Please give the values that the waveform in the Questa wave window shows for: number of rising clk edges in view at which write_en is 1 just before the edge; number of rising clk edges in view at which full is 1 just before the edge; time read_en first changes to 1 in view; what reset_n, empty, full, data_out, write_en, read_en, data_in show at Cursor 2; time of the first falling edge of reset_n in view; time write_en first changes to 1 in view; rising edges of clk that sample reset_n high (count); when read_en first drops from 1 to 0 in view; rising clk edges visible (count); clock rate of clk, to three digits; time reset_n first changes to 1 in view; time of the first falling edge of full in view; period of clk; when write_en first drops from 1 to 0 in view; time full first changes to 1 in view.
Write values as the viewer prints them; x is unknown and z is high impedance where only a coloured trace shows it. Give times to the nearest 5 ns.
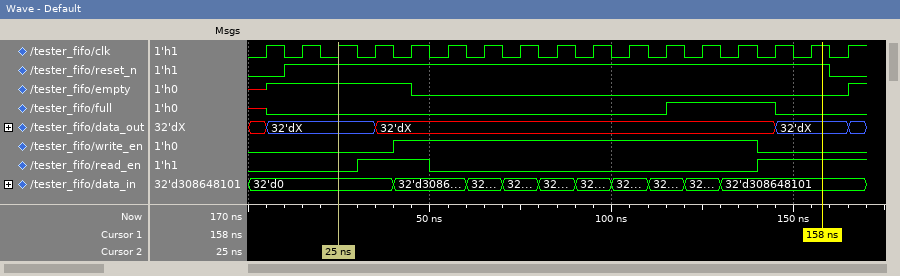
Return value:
10
3
30 ns
reset_n=1, empty=1, full=0, data_out=32'dX, write_en=0, read_en=0, data_in=32'd0
160 ns
40 ns
15
50 ns
17
100 MHz
10 ns
145 ns
10 ns
140 ns
115 ns
